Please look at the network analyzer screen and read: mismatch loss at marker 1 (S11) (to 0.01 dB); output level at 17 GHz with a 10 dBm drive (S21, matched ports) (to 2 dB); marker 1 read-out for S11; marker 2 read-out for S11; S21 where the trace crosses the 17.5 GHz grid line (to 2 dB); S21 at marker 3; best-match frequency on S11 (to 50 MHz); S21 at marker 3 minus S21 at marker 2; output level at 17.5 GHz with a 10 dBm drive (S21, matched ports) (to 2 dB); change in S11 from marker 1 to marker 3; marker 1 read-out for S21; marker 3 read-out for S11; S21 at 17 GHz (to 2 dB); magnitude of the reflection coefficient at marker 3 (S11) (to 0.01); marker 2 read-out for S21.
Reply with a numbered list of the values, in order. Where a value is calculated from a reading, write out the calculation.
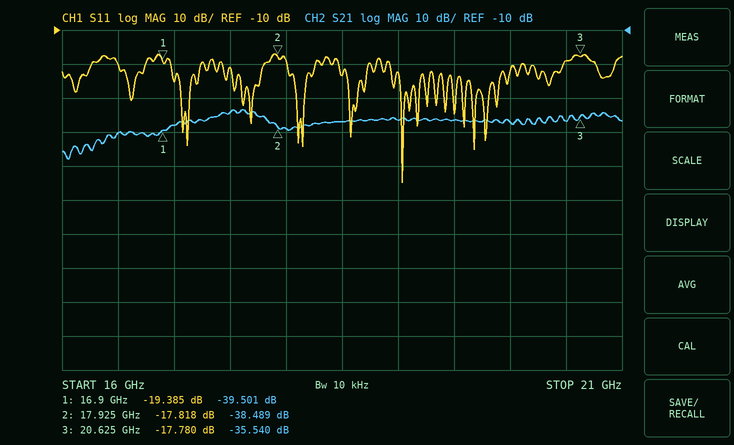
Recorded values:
1. −10 log10(1 − 10^(-19.385/10)) ≈ 0.05 dB
2. 10 dBm + (-38 dB) = -28 dBm
3. -19.385 dB
4. -17.818 dB
5. -34 dB
6. -35.540 dB
7. 19.05 GHz
8. -35.54 − (-38.489) = 2.949 dB
9. 10 dBm + (-34 dB) = -24 dBm
10. -17.78 − (-19.385) = 1.605 dB
11. -39.501 dB
12. -17.780 dB
13. -38 dB
14. 10^(-17.78/20) ≈ 0.13
15. -38.489 dB
